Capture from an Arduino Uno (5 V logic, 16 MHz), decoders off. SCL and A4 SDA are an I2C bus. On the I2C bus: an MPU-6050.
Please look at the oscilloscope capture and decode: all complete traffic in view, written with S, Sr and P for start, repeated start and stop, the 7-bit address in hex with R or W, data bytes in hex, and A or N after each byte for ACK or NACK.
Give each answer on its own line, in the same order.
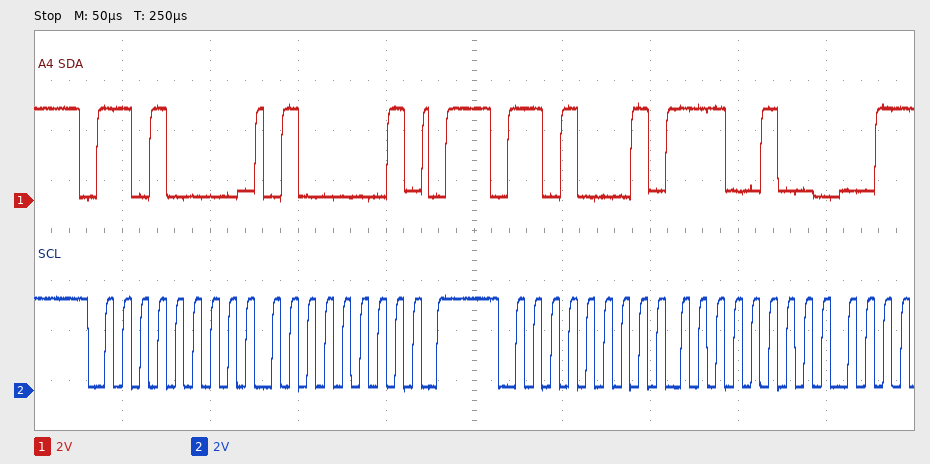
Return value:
S 68W A 41 A P S 68R A E4 A
